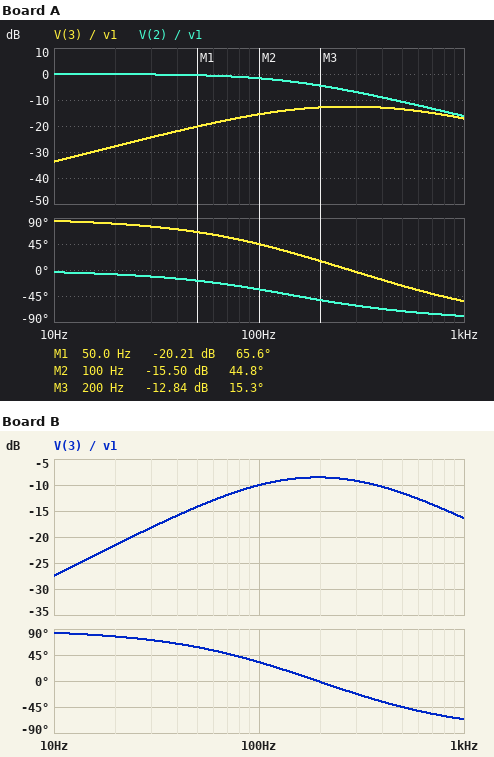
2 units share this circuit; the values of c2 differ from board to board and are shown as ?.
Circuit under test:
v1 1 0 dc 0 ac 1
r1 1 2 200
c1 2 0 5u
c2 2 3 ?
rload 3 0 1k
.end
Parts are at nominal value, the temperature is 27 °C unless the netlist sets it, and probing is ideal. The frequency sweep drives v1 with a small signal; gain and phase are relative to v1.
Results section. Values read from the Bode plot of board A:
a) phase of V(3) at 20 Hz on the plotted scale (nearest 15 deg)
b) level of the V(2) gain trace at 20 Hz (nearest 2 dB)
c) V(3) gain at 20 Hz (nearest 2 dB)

75 deg
0 dB
-28 dB
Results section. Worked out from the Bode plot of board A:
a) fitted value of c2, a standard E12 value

330 nF
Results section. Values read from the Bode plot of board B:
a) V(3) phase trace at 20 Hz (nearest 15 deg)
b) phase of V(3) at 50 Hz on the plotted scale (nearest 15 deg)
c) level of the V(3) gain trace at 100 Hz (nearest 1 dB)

75 deg
60 deg
-10 dB
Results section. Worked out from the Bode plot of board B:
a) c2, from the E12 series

680 nF
